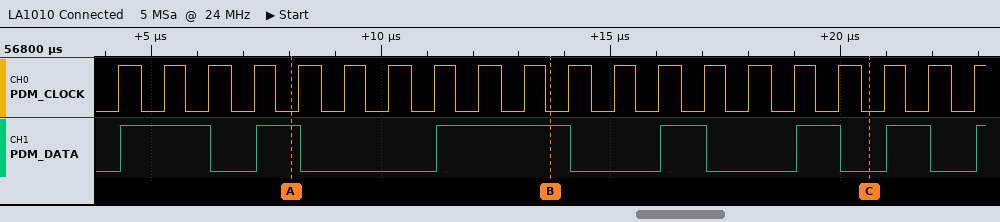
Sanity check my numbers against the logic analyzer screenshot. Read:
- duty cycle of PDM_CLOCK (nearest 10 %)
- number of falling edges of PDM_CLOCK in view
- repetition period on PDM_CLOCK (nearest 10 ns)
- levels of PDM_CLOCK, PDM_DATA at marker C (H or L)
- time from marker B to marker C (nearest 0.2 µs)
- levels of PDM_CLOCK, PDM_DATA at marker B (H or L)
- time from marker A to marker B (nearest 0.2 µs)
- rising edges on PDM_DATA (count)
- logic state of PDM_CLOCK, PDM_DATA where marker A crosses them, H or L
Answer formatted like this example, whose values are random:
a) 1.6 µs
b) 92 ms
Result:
a) 50 %
b) 19
c) 980 ns
d) PDM_CLOCK=L, PDM_DATA=L
e) 7 µs
f) PDM_CLOCK=L, PDM_DATA=H
g) 5.6 µs
h) 7
i) PDM_CLOCK=L, PDM_DATA=H
